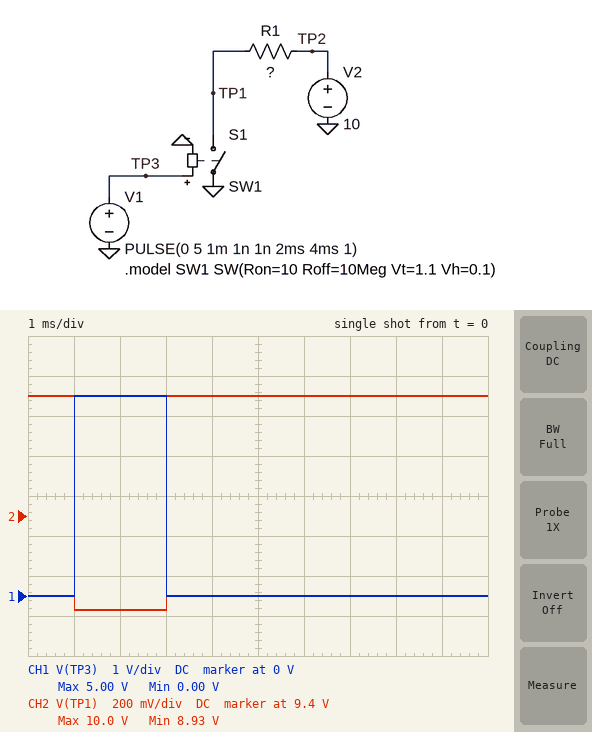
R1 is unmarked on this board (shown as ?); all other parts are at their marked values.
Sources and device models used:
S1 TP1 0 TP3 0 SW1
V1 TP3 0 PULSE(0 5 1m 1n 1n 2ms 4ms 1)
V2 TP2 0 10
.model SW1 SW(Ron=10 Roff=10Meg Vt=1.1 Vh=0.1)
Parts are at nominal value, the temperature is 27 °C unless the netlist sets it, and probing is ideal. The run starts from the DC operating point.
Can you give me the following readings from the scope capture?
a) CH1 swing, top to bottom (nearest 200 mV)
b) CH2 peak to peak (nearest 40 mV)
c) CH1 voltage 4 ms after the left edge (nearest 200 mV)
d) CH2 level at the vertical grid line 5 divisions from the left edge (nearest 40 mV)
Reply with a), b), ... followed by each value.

a) 5.0 V
b) 1.08 V
c) 0 V
d) 10.00 V
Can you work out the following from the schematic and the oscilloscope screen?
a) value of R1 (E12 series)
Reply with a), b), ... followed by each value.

a) 1.2 Ω
